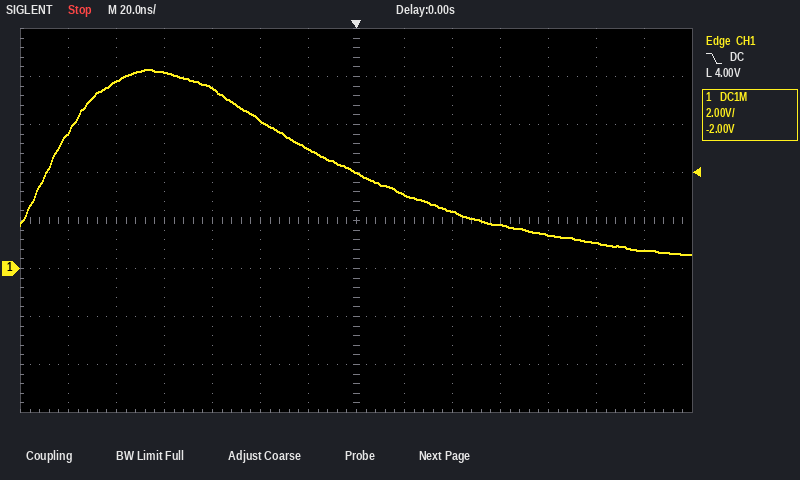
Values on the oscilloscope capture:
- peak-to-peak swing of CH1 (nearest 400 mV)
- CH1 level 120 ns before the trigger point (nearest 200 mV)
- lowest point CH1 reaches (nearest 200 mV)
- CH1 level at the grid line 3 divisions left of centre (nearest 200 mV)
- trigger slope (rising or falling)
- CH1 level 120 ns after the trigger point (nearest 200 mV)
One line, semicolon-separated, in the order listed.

7.6 V; 5.6 V; 600 mV; 7.6 V; falling; 800 mV
